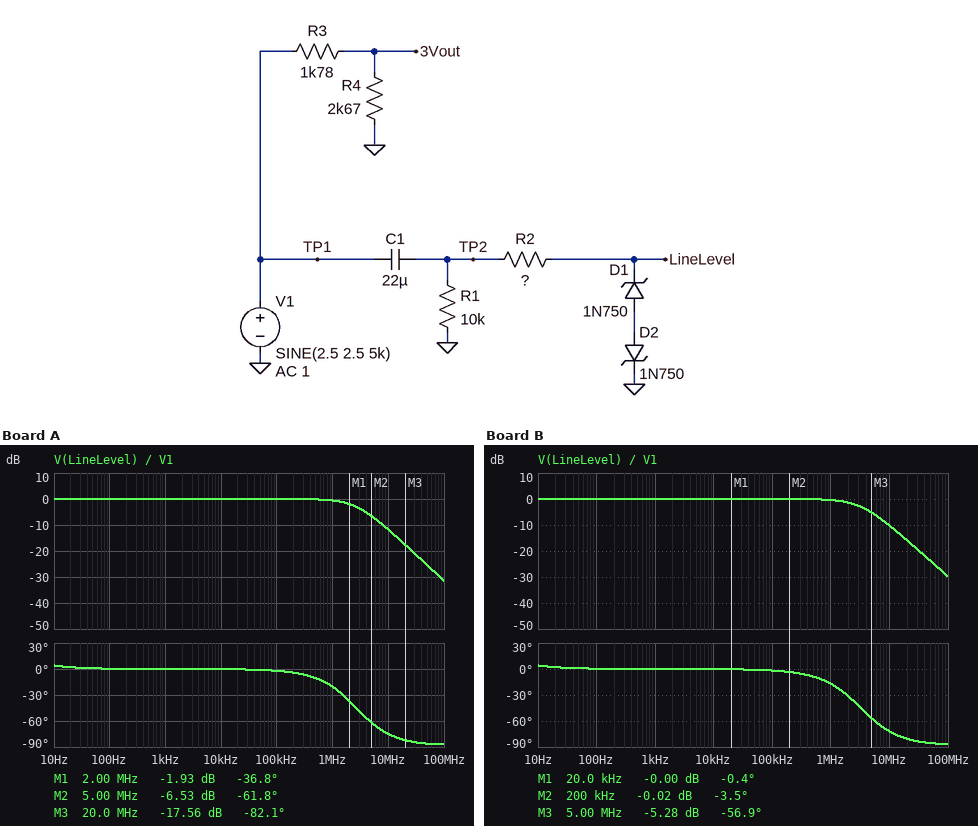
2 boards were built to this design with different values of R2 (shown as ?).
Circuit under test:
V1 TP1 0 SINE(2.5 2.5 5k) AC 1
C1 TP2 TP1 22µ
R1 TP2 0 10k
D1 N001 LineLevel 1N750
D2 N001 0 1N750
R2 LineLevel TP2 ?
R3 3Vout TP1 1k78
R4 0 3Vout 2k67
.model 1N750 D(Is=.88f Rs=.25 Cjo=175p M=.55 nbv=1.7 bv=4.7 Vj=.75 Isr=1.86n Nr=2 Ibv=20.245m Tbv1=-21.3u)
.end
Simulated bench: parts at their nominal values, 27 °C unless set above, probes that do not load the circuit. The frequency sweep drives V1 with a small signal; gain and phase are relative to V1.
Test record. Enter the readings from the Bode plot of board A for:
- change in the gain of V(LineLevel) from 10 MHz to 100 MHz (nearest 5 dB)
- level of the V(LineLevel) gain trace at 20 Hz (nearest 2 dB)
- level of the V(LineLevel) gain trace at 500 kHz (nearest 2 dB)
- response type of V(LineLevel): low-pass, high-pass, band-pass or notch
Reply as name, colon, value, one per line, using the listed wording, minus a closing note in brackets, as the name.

change in the gain of V(LineLevel) from 10 MHz to 100 MHz: -20 dB
level of the V(LineLevel) gain trace at 20 Hz: 0 dB
level of the V(LineLevel) gain trace at 500 kHz: 0 dB
response type of V(LineLevel): low-pass, high-pass, band-pass or notch: low-pass
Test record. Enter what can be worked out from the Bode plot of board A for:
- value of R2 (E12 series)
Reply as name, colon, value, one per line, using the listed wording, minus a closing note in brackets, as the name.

value of R2: 680 Ω
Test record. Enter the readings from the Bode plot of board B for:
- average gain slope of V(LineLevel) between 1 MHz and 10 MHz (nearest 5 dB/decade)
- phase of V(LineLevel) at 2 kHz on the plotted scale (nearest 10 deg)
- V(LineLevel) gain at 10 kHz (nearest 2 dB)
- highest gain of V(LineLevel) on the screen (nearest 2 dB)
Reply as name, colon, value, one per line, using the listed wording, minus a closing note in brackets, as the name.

average gain slope of V(LineLevel) between 1 MHz and 10 MHz: -10 dB/decade
phase of V(LineLevel) at 2 kHz on the plotted scale: 0 deg
V(LineLevel) gain at 10 kHz: 0 dB
highest gain of V(LineLevel) on the screen: 0 dB
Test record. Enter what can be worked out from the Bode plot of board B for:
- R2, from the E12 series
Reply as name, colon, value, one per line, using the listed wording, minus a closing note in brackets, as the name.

R2, from the E12 series: 560 Ω
